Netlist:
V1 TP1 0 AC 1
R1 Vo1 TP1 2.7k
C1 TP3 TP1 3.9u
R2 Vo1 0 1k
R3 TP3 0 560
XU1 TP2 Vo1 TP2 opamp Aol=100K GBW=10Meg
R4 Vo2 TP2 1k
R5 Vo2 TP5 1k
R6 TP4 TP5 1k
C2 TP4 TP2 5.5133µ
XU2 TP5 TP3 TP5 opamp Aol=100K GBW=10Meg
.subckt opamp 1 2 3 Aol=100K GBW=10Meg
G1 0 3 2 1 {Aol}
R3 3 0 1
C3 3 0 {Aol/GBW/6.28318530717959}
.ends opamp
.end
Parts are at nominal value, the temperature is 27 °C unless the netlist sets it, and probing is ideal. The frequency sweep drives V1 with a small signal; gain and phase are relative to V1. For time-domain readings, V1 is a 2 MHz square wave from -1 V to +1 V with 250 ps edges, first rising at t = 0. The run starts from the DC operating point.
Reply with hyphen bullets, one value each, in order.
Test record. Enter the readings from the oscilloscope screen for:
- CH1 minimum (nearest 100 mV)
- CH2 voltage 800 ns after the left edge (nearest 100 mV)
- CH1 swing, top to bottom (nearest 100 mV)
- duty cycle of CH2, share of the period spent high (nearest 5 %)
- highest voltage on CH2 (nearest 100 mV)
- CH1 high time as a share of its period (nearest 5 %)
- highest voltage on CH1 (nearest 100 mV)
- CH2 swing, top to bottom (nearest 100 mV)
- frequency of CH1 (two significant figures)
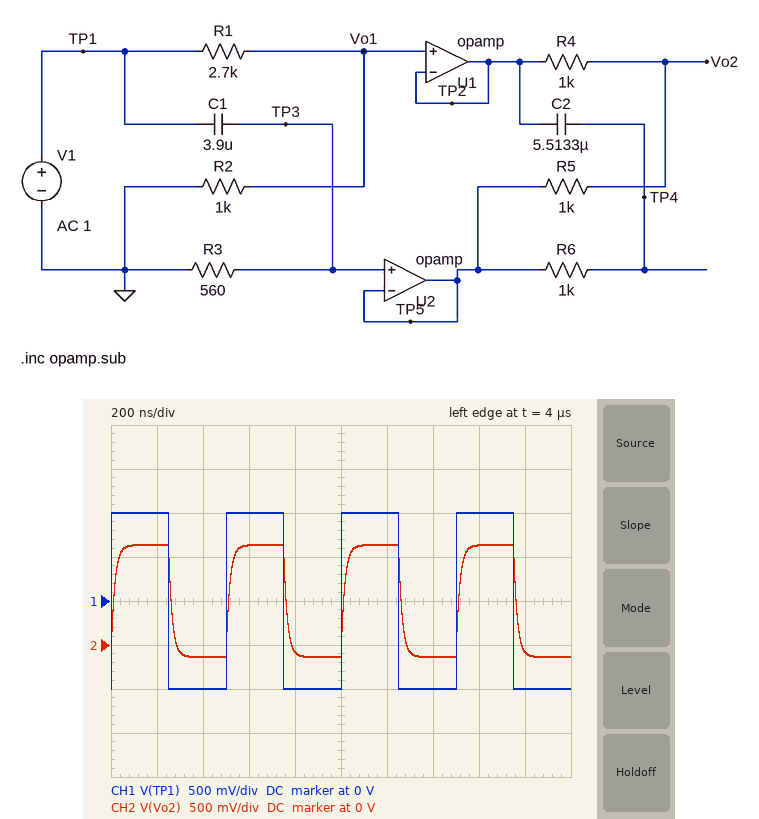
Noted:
- -1.0 V
- -100 mV
- 2.0 V
- 50 %
- 1.1 V
- 50 %
- 1.0 V
- 1.3 V
- 2.0 MHz
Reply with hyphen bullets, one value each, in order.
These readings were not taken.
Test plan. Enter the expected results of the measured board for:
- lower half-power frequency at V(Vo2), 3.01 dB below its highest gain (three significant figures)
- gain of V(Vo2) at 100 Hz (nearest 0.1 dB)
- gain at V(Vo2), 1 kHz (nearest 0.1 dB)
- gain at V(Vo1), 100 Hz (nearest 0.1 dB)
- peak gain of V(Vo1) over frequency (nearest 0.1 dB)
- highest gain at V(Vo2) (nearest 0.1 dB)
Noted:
- 69.5 Hz
- -5.7 dB
- -4.0 dB
- -11.4 dB
- -11.4 dB
- -3.9 dB
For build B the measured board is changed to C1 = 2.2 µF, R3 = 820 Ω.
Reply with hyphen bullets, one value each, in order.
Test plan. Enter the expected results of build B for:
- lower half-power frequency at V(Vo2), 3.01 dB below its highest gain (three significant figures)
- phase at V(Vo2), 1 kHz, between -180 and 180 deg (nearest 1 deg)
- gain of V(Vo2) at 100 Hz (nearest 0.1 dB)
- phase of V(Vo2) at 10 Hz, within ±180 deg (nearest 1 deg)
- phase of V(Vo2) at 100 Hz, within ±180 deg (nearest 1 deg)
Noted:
- 84.1 Hz
- 4 deg
- -6.3 dB
- 22 deg
- 31 deg
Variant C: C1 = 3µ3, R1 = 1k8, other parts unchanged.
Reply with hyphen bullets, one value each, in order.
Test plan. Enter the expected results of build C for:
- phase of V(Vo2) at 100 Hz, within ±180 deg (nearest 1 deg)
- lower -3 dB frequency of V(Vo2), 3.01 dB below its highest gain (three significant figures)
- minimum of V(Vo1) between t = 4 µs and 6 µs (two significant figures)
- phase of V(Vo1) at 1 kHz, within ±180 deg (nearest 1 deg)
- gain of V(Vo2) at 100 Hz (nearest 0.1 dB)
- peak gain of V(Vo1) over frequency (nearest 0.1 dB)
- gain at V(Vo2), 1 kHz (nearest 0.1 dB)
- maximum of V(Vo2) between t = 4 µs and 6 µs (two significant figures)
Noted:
- 28 deg
- 79.9 Hz
- -360 mV
- 0 deg
- -5.6 dB
- -8.9 dB
- -3.4 dB
- 1.2 V
